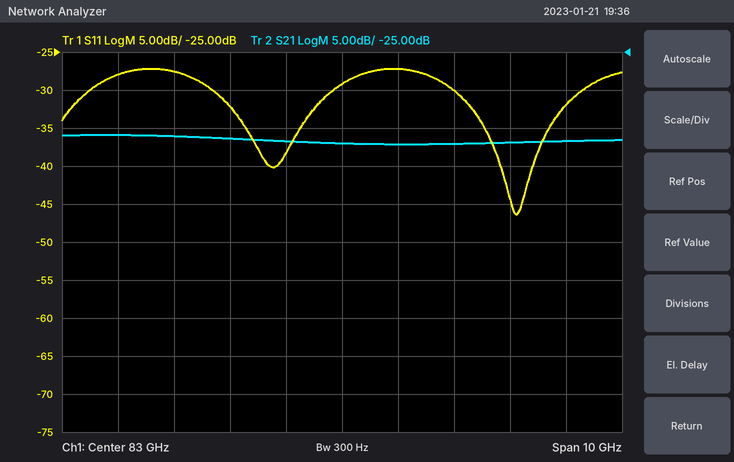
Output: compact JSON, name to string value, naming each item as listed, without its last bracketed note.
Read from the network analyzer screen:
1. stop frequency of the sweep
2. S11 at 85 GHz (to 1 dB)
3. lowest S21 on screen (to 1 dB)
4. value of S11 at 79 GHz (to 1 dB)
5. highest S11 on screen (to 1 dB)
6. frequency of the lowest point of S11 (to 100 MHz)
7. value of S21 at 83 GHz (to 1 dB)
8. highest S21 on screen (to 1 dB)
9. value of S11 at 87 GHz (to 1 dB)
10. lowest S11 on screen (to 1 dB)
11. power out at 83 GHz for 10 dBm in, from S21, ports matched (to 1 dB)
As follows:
{"stop frequency of the sweep": "88 GHz", "S11 at 85 GHz": "-30 dB", "lowest S21 on screen": "-37 dB", "value of S11 at 79 GHz": "-28 dB", "highest S11 on screen": "-27 dB", "frequency of the lowest point of S11": "86.1 GHz", "value of S21 at 83 GHz": "-37 dB", "highest S21 on screen": "-36 dB", "value of S11 at 87 GHz": "-32 dB", "lowest S11 on screen": "-46 dB", "power out at 83 GHz for 10 dBm in, from S21, ports matched": "-27 dBm"}
